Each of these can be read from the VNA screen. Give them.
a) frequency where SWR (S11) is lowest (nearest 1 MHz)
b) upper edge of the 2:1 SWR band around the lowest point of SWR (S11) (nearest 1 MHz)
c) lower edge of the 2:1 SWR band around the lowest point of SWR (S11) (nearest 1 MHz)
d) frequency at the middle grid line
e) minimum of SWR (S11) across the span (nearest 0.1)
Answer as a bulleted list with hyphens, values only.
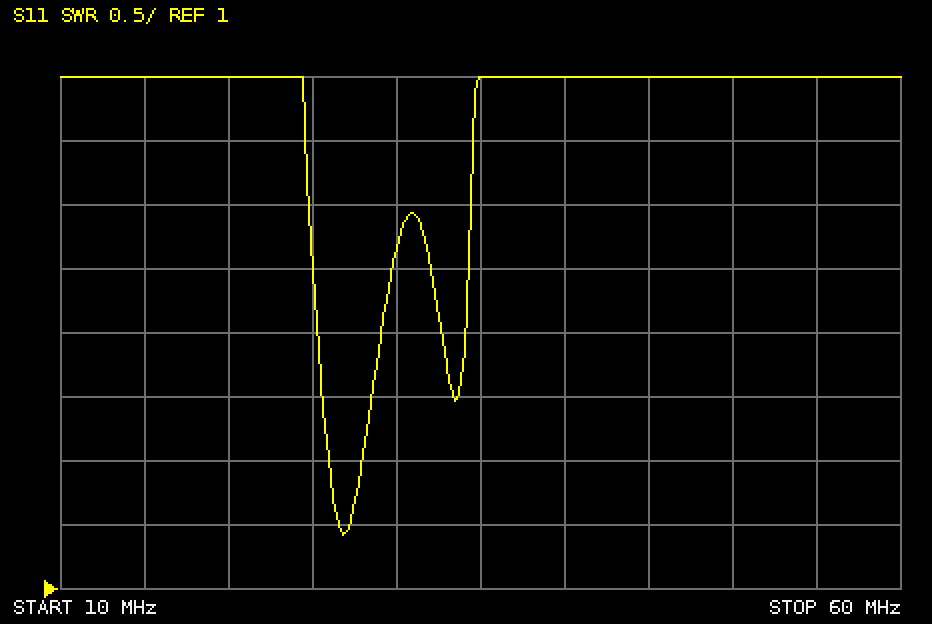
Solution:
- 27 MHz
- 28 MHz
- 26 MHz
- 35 MHz
- 1.4
